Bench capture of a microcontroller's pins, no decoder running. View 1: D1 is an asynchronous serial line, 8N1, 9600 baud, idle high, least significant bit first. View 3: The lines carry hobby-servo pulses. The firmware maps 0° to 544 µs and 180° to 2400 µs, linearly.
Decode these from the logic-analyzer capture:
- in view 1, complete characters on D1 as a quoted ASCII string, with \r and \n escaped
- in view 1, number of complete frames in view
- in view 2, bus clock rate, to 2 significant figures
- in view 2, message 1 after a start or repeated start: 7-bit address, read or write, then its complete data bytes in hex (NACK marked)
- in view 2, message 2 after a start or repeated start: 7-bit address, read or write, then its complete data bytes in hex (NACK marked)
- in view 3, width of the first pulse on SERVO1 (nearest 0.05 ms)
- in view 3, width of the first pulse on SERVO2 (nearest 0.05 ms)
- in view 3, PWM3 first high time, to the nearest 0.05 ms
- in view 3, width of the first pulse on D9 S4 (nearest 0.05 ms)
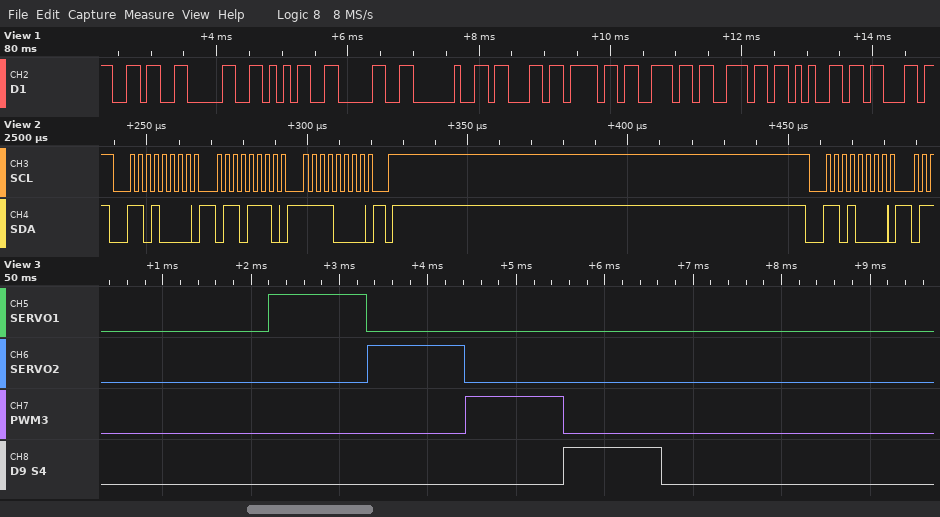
"6050 connec"
11
400 kHz
0x68 write: 6E F0
0x68 write
1.10 ms
1.10 ms
1.10 ms
1.10 ms
